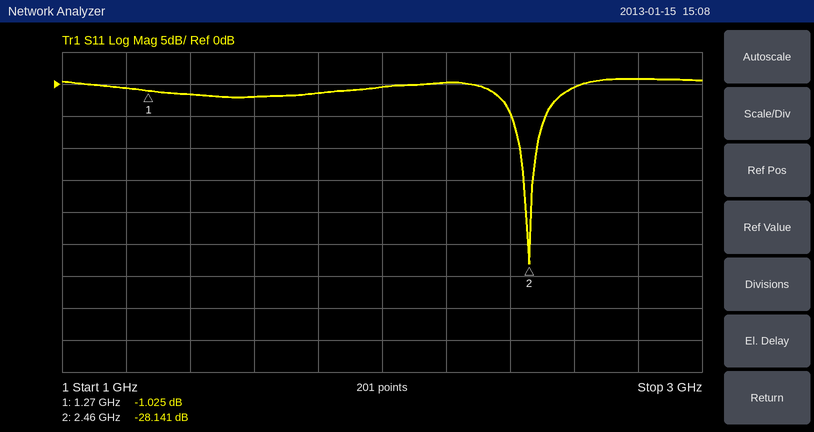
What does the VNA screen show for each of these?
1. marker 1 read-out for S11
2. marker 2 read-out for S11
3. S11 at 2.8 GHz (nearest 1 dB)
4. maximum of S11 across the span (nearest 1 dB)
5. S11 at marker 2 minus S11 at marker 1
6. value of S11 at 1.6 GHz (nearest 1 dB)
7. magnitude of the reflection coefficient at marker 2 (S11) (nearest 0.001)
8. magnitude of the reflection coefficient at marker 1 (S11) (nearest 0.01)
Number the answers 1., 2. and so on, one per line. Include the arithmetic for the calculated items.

1. -1.025 dB
2. -28.141 dB
3. 1 dB
4. 1 dB
5. -28.141 − (-1.025) = -27.116 dB
6. -2 dB
7. 10^(-28.141/20) ≈ 0.039
8. 10^(-1.025/20) ≈ 0.89
